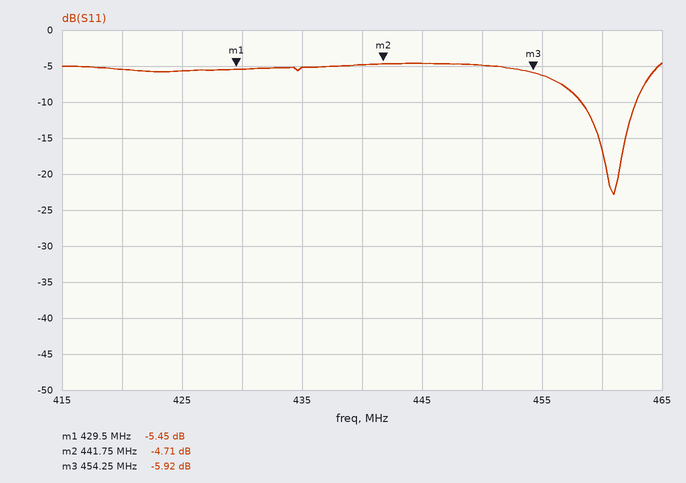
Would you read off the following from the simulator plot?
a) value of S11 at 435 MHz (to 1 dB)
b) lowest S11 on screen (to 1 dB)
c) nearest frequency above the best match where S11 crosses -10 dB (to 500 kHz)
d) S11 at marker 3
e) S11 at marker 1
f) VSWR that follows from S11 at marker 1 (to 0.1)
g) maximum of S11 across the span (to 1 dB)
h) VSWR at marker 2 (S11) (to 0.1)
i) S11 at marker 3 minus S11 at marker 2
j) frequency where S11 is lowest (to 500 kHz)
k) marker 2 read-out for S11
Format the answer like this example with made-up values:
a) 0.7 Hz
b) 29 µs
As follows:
a) -5 dB
b) -23 dB
c) 463.0 MHz
d) -5.92 dB
e) -5.45 dB
f) 3.3
g) -5 dB
h) 3.8
i) -1.21 dB
j) 461.0 MHz
k) -4.71 dB
